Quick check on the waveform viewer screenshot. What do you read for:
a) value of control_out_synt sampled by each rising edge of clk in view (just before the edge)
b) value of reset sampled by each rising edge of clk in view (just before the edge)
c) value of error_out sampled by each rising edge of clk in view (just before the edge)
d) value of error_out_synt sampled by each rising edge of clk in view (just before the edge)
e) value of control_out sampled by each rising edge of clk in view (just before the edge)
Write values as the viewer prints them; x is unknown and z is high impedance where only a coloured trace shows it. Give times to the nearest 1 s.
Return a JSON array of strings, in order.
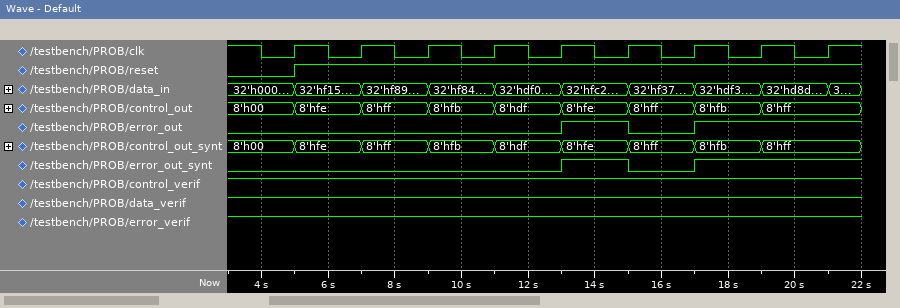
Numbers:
["8'h00, 8'hfe, 8'hff, 8'hfb, 8'hdf, 8'hfe, 8'hff, 8'hfb, 8'hff", "0 1 1 1 1 1 1 1 1", "0 0 0 0 0 1 0 1 1", "0 0 0 0 0 1 0 1 1", "8'h00, 8'hfe, 8'hff, 8'hfb, 8'hdf, 8'hfe, 8'hff, 8'hfb, 8'hff"]
